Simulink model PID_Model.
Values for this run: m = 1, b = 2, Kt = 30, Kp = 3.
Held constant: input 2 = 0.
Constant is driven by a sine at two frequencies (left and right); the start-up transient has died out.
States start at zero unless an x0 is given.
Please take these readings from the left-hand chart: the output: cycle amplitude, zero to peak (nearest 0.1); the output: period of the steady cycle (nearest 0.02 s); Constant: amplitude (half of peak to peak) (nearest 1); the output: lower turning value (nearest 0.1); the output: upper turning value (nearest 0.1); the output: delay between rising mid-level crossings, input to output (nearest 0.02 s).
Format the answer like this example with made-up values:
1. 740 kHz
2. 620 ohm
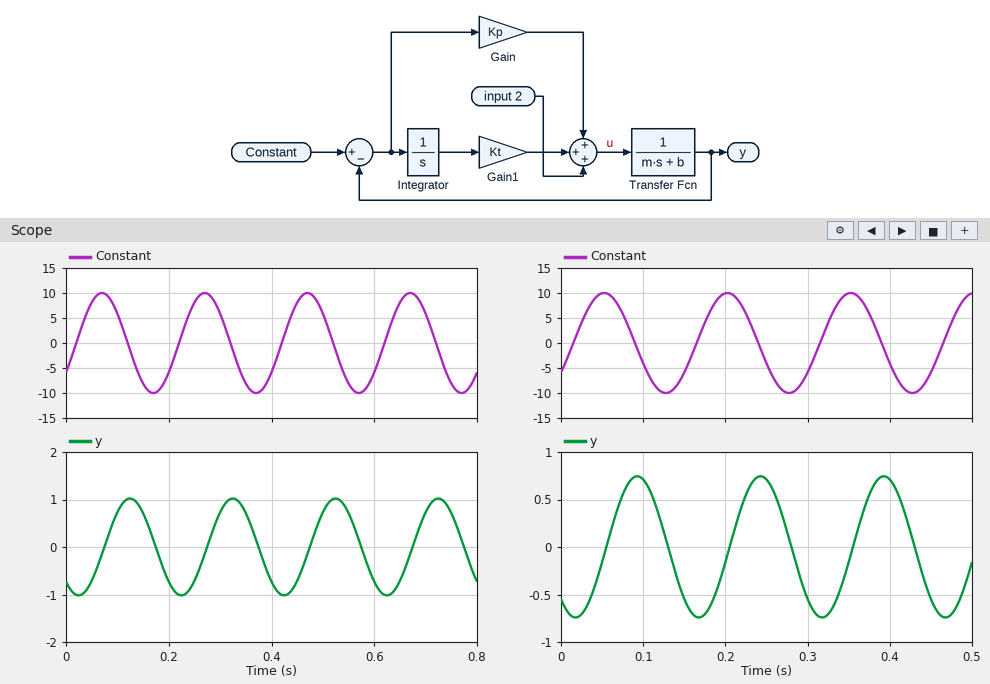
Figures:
1. 1.0
2. 0.20 s
3. 10
4. -1.0
5. 1.0
6. 0.06 s
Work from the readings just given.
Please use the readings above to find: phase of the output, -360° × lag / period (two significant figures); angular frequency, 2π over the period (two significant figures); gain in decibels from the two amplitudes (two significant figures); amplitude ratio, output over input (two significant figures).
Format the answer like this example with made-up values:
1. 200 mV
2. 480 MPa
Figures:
1. -110°
2. 31 rad/s
3. -20 dB
4. 0.10
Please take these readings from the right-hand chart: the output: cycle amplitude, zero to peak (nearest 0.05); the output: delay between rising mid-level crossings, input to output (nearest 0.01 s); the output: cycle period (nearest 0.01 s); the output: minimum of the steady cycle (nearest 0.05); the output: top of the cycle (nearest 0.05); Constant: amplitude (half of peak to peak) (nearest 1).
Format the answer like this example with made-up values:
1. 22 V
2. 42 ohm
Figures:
1. 0.75
2. 0.04 s
3. 0.15 s
4. -0.75
5. 0.75
6. 10
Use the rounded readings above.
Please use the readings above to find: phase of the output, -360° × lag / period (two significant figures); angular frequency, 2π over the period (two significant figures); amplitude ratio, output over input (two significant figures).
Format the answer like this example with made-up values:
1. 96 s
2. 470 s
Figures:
1. -96°
2. 42 rad/s
3. 0.075
